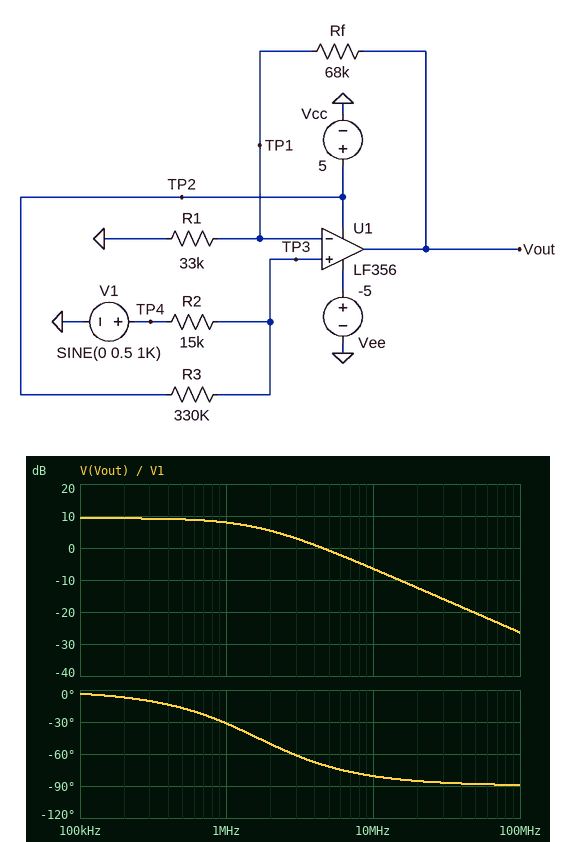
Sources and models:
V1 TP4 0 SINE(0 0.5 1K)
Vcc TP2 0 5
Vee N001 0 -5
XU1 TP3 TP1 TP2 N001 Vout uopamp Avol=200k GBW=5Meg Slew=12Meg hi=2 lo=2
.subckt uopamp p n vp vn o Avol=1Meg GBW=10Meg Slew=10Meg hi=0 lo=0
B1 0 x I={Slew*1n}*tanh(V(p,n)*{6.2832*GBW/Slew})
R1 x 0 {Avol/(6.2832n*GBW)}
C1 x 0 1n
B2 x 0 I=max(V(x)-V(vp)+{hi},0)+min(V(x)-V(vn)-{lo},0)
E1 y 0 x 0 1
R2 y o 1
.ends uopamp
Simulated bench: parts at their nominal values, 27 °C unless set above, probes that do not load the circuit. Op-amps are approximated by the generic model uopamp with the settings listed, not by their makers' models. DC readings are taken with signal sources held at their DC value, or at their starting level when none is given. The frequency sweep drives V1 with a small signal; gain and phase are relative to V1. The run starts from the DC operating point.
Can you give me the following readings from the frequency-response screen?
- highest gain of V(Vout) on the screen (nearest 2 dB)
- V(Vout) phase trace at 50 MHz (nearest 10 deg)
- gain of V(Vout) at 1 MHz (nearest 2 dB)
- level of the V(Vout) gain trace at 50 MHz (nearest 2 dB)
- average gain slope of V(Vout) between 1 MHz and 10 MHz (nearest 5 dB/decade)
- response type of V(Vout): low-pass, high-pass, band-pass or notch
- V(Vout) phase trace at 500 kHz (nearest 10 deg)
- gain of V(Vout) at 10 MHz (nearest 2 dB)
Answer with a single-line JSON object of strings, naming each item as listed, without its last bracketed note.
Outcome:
{"highest gain of V(Vout) on the screen": "10 dB", "V(Vout) phase trace at 50 MHz": "-90 deg", "gain of V(Vout) at 1 MHz": "8 dB", "level of the V(Vout) gain trace at 50 MHz": "-20 dB", "average gain slope of V(Vout) between 1 MHz and 10 MHz": "-15 dB/decade", "response type of V(Vout): low-pass, high-pass, band-pass or notch": "low-pass", "V(Vout) phase trace at 500 kHz": "-20 deg", "gain of V(Vout) at 10 MHz": "-6 dB"}
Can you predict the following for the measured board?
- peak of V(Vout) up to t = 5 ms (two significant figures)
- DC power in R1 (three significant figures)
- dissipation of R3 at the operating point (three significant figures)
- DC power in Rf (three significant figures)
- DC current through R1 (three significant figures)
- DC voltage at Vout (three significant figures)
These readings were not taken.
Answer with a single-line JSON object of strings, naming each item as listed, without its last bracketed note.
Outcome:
{"peak of V(Vout) up to t = 5 ms": "2.1 V", "DC power in R1": "1.43 µW", "dissipation of R3 at the operating point": "69.3 µW", "DC power in Rf": "2.95 µW", "DC current through R1": "6.59 µA", "DC voltage at Vout": "665 mV"}
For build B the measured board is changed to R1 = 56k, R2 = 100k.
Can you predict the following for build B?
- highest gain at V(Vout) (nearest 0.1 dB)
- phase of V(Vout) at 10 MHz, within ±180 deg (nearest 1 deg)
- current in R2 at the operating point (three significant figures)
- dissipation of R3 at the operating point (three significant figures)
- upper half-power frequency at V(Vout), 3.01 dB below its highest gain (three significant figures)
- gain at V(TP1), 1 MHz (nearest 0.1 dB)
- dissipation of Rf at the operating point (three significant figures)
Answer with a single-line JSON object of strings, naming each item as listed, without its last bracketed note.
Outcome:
{"highest gain at V(Vout)": "4.6 dB", "phase of V(Vout) at 10 MHz, within ±180 deg": "-77 deg", "current in R2 at the operating point": "11.6 µA", "dissipation of R3 at the operating point": "44.6 µW", "upper half-power frequency at V(Vout), 3.01 dB below its highest gain": "2.26 MHz", "gain at V(TP1), 1 MHz": "-3.1 dB", "dissipation of Rf at the operating point": "29.3 µW"}
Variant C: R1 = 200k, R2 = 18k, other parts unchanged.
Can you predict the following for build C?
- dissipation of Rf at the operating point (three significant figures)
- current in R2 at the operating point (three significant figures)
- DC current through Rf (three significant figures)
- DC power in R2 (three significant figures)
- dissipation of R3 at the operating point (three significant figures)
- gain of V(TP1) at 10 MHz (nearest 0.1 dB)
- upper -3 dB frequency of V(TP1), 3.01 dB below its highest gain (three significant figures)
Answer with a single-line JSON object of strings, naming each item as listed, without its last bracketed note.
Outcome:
{"dissipation of Rf at the operating point": "114 nW", "current in R2 at the operating point": "14.4 µA", "DC current through Rf": "1.29 µA", "DC power in R2": "3.72 µW", "dissipation of R3 at the operating point": "68.1 µW", "gain of V(TP1) at 10 MHz": "-9.6 dB", "upper -3 dB frequency of V(TP1), 3.01 dB below its highest gain": "3.73 MHz"}
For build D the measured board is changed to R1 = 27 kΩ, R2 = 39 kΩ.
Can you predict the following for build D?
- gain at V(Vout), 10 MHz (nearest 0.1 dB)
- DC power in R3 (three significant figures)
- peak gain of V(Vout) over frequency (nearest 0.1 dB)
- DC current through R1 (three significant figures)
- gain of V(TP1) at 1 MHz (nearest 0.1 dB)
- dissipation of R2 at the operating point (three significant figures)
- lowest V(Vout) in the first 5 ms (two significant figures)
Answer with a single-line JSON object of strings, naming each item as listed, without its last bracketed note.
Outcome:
{"gain at V(Vout), 10 MHz": "-7.1 dB", "DC power in R3": "60.6 µW", "peak gain of V(Vout) over frequency": "10.0 dB", "DC current through R1": "19.6 µA", "gain of V(TP1) at 1 MHz": "-2.7 dB", "dissipation of R2 at the operating point": "7.16 µW", "lowest V(Vout) in the first 5 ms": "290 mV"}
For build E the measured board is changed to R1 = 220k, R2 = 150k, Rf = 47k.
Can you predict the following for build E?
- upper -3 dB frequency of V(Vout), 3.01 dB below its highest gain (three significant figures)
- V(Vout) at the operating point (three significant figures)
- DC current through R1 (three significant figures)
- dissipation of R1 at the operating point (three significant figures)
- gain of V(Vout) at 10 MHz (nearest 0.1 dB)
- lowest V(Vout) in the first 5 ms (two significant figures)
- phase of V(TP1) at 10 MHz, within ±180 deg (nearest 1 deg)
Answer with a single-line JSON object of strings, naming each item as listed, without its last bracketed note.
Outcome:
{"upper -3 dB frequency of V(Vout), 3.01 dB below its highest gain": "4.12 MHz", "V(Vout) at the operating point": "1.90 V", "DC current through R1": "7.10 µA", "dissipation of R1 at the operating point": "11.1 µW", "gain of V(Vout) at 10 MHz": "-10.0 dB", "lowest V(Vout) in the first 5 ms": "1.5 V", "phase of V(TP1) at 10 MHz, within ±180 deg": "-68 deg"}
